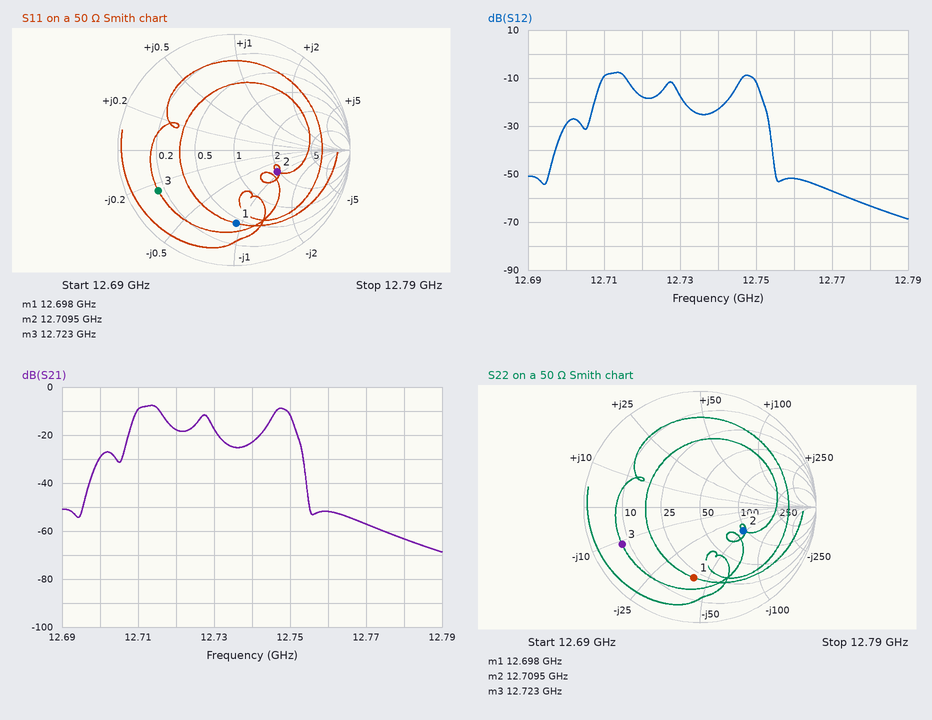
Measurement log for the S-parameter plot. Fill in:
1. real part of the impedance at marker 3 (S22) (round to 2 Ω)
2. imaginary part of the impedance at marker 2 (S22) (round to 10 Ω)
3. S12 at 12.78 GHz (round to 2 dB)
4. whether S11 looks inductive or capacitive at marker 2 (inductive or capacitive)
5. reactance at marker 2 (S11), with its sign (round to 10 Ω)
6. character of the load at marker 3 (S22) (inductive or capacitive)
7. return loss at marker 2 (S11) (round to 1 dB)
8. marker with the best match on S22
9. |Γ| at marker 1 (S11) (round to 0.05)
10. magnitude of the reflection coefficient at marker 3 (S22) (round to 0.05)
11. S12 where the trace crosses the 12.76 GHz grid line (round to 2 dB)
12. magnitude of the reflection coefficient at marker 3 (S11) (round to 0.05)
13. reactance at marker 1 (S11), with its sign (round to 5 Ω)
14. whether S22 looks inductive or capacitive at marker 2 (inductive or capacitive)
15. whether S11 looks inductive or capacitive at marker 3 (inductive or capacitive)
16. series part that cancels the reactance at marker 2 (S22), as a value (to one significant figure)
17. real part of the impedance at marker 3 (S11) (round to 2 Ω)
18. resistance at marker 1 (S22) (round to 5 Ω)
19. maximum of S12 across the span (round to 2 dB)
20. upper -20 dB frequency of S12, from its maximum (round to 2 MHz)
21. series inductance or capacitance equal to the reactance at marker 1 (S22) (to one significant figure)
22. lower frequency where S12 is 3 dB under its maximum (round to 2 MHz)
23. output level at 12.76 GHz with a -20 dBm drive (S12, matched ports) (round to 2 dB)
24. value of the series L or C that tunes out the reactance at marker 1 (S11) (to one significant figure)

8 Ω
-50 Ω
-64 dB
capacitive
-40 Ω
capacitive
8 dB
marker 2
0.65
0.75
-52 dB
0.75
-45 Ω
capacitive
capacitive
600 pH
8 Ω
20 Ω
-8 dB
12.754 GHz
300 fF
12.710 GHz
-72 dBm
600 pH
